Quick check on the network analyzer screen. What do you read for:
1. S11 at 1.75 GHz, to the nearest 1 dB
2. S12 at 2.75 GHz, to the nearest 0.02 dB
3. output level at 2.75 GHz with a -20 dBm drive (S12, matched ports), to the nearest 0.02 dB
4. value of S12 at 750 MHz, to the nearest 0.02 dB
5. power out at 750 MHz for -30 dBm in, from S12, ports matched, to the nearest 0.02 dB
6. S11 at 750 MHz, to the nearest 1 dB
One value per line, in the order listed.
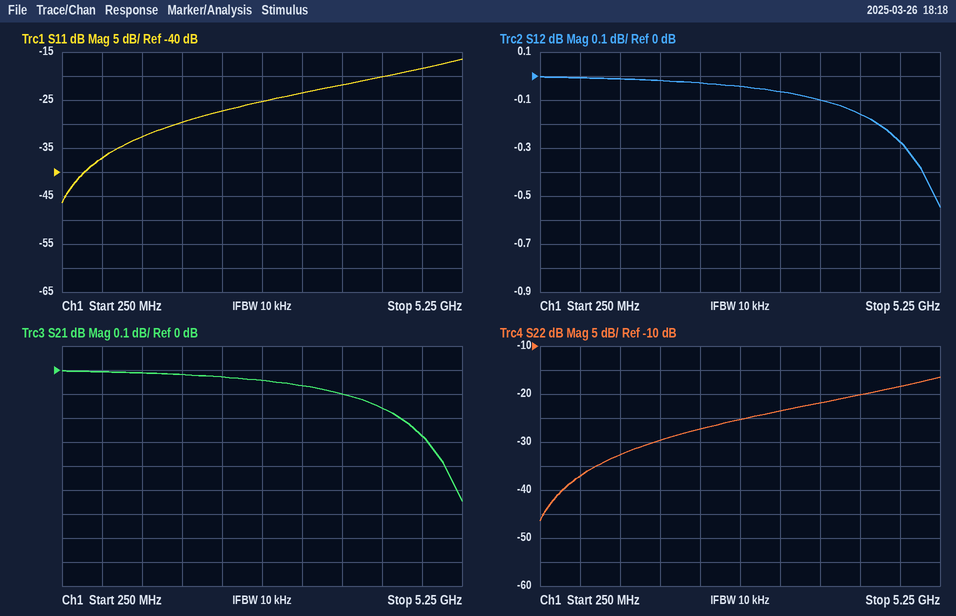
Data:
-30 dB
-0.04 dB
-20.04 dBm
0.00 dB
-30.00 dBm
-37 dB
